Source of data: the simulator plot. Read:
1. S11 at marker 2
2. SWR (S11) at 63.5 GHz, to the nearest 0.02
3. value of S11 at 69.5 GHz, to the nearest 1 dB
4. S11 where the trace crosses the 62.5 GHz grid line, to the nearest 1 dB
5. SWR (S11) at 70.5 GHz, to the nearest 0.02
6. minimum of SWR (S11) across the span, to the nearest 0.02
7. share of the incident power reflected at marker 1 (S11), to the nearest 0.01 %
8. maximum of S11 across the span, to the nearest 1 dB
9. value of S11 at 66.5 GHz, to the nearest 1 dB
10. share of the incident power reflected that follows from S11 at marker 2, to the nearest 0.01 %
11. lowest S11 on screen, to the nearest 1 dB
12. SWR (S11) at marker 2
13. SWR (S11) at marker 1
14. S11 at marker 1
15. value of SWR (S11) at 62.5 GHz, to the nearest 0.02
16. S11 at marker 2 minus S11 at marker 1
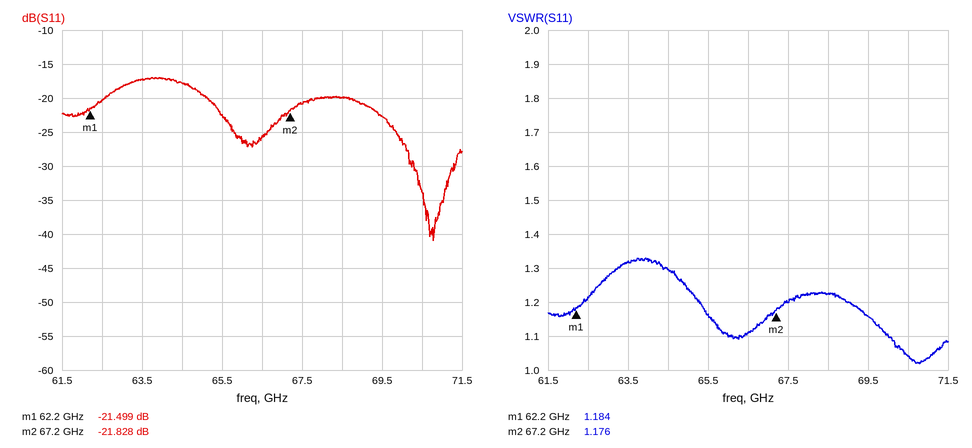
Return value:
-21.828 dB
1.32
-23 dB
-20 dB
1.04
1.02
0.71 %
-17 dB
-26 dB
0.66 %
-41 dB
1.176
1.184
-21.499 dB
1.22
-0.329 dB
